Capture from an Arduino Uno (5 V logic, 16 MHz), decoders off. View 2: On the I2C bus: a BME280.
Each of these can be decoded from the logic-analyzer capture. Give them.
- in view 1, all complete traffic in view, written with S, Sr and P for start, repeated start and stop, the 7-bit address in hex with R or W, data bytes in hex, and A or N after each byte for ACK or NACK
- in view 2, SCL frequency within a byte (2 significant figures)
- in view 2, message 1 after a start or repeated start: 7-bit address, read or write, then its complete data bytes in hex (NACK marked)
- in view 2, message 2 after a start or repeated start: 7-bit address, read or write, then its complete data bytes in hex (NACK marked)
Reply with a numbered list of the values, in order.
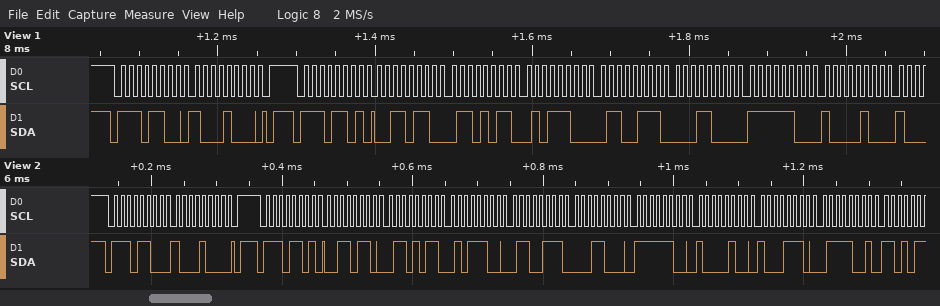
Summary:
1. S 76W A 88 A P S 76R A 36 A 6B A 5C A 67 A 18 A FC A 84 A
2. 100 kHz
3. 0x76 write: 88
4. 0x76 read: 36 6B 5C 67 18 FC 84 8E 79
